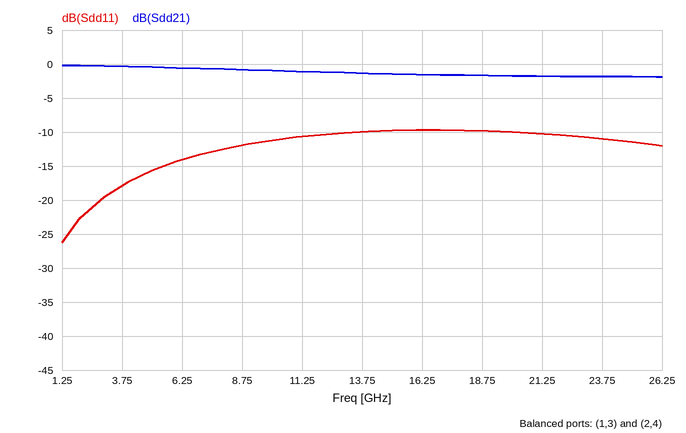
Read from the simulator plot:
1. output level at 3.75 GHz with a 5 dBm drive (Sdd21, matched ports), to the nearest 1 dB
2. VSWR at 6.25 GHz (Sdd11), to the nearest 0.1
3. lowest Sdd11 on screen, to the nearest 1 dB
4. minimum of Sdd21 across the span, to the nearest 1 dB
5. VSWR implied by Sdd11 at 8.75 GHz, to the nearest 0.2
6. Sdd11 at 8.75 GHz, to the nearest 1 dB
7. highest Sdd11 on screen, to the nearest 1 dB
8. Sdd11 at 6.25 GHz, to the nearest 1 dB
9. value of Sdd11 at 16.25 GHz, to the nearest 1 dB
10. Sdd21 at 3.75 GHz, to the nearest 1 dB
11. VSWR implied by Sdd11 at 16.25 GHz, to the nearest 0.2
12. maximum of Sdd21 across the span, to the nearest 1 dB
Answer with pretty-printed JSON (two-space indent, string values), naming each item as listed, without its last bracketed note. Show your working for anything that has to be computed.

{
  "output level at 3.75 GHz with a 5 dBm drive (Sdd21, matched ports), to the nearest 1 dB": "5 dBm + (0 dB) = 5 dBm",
  "VSWR at 6.25 GHz (Sdd11), to the nearest 0.1": "|Γ| = 10^(-14/20) = 0.1995; VSWR = (1 + 0.1995)/(1 − 0.1995) ≈ 1.5",
  "lowest Sdd11 on screen, to the nearest 1 dB": "-26 dB",
  "minimum of Sdd21 across the span, to the nearest 1 dB": "-2 dB",
  "VSWR implied by Sdd11 at 8.75 GHz, to the nearest 0.2": "|Γ| = 10^(-12/20) = 0.2512; VSWR = (1 + 0.2512)/(1 − 0.2512) ≈ 1.67, so 1.6 to the nearest 0.2",
  "Sdd11 at 8.75 GHz, to the nearest 1 dB": "-12 dB",
  "highest Sdd11 on screen, to the nearest 1 dB": "-10 dB",
  "Sdd11 at 6.25 GHz, to the nearest 1 dB": "-14 dB",
  "value of Sdd11 at 16.25 GHz, to the nearest 1 dB": "-10 dB",
  "Sdd21 at 3.75 GHz, to the nearest 1 dB": "0 dB",
  "VSWR implied by Sdd11 at 16.25 GHz, to the nearest 0.2": "|Γ| = 10^(-10/20) = 0.3162; VSWR = (1 + 0.3162)/(1 − 0.3162) ≈ 1.92, so 2.0 to the nearest 0.2",
  "maximum of Sdd21 across the span, to the nearest 1 dB": "0 dB"
}
